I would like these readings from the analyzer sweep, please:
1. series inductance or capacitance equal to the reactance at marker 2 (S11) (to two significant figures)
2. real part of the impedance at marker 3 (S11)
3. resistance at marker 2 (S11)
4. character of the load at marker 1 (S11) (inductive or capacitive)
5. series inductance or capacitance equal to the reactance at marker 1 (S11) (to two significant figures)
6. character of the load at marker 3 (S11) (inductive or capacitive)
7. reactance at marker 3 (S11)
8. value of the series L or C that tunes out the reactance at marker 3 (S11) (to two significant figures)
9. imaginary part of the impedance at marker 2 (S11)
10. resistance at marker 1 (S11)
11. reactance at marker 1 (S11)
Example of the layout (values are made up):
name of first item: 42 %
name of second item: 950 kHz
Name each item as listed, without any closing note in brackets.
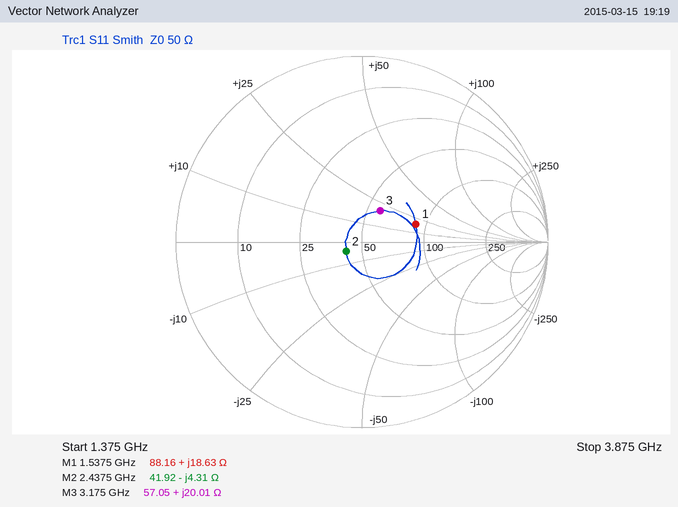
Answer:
series inductance or capacitance equal to the reactance at marker 2 (S11): 15 pF
real part of the impedance at marker 3: 57.05 Ω
resistance at marker 2: 41.92 Ω
character of the load at marker 1 (S11): inductive
series inductance or capacitance equal to the reactance at marker 1 (S11): 1.9 nH
character of the load at marker 3 (S11): inductive
reactance at marker 3: +20.01 Ω
value of the series L or C that tunes out the reactance at marker 3 (S11): 2.5 pF
imaginary part of the impedance at marker 2: -4.31 Ω
resistance at marker 1: 88.16 Ω
reactance at marker 1: +18.63 Ω
